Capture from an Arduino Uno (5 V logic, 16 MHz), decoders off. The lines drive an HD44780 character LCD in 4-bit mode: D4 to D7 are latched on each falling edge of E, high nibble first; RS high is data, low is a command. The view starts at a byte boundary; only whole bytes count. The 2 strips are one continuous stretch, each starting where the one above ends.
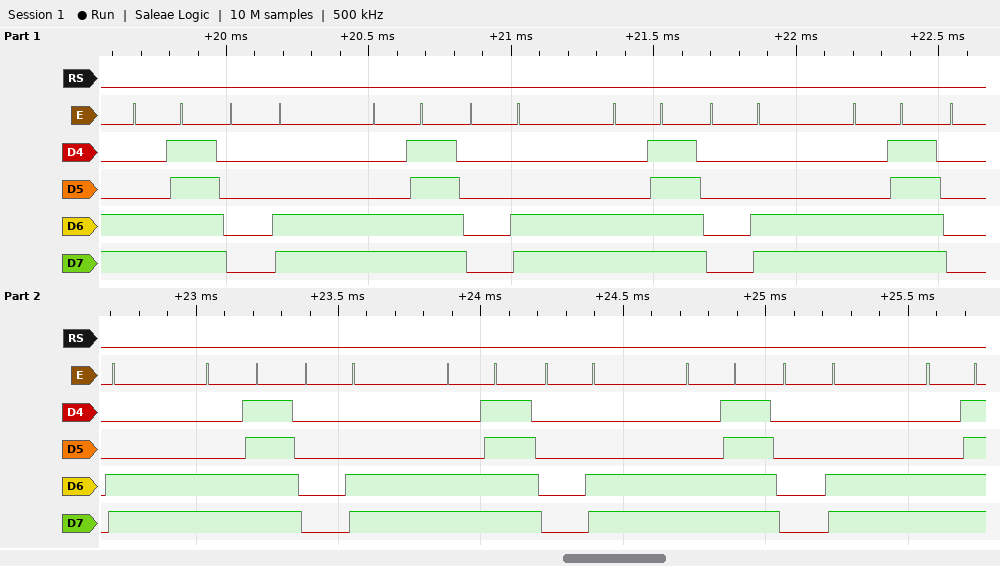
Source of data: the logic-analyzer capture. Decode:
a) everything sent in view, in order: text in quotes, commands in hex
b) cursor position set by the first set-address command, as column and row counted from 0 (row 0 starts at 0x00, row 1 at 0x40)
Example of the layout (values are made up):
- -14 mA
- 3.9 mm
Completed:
- 0xCF 0x0C 0xCF 0x0C 0xCF 0x0C 0xCF 0x0C 0xCF 0x0C 0xCF 0x0C 0xCF 0x0C 0xCF
- column 15, row 1
